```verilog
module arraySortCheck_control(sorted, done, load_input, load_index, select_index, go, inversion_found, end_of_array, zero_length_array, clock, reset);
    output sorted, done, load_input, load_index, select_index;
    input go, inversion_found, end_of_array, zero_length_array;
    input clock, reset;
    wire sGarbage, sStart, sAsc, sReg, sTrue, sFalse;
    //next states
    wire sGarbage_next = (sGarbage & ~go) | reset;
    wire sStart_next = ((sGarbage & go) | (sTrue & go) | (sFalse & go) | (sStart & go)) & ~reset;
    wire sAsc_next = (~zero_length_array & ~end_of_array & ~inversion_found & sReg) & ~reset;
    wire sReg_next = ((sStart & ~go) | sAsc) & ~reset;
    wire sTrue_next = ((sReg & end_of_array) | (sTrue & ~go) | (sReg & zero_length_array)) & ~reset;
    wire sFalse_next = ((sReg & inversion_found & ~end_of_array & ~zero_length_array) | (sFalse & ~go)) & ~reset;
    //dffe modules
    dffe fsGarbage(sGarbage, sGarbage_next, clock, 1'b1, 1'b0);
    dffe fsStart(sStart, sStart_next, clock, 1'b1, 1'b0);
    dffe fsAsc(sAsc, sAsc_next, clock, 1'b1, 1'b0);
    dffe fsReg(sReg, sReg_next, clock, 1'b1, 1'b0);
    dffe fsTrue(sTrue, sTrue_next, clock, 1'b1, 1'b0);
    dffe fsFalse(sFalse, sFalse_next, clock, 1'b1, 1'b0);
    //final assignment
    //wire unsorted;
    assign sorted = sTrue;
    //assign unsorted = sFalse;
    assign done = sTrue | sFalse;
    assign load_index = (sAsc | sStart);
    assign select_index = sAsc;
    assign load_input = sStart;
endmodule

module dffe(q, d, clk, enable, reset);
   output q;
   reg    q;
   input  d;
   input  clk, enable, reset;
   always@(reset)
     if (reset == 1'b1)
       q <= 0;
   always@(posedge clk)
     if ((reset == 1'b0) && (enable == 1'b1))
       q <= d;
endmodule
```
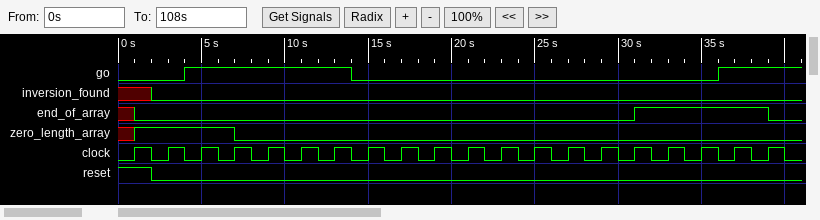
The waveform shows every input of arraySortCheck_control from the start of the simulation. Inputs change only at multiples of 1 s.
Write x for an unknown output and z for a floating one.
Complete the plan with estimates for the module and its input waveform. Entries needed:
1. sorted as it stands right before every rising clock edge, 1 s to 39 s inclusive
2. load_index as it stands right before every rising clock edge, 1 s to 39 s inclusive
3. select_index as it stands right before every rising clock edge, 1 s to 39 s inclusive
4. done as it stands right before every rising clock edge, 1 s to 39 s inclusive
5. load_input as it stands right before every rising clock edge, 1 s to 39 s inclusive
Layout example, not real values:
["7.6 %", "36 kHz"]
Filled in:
["x 0 0 0 0 0 0 0 0 0 0 0 0 0 0 0 0 1 1 0", "x 0 0 1 1 1 1 1 0 1 0 1 0 1 0 1 0 0 0 1", "x 0 0 0 0 0 0 0 0 1 0 1 0 1 0 1 0 0 0 0", "x 0 0 0 0 0 0 0 0 0 0 0 0 0 0 0 0 1 1 0", "x 0 0 1 1 1 1 1 0 0 0 0 0 0 0 0 0 0 0 1"]
